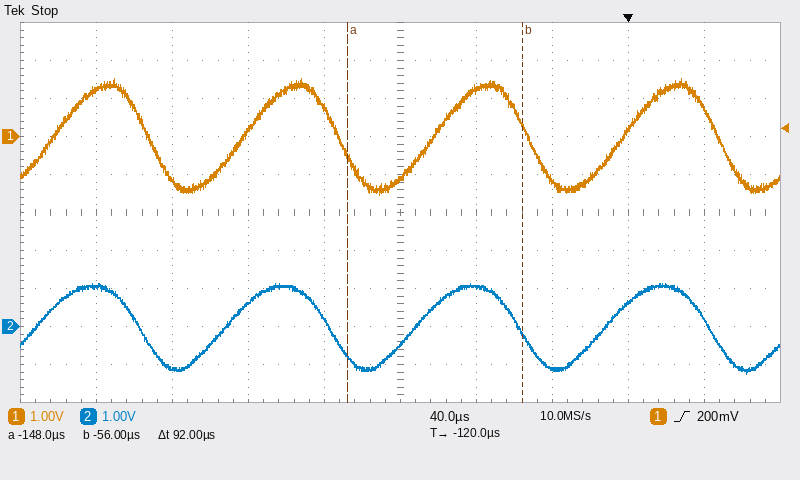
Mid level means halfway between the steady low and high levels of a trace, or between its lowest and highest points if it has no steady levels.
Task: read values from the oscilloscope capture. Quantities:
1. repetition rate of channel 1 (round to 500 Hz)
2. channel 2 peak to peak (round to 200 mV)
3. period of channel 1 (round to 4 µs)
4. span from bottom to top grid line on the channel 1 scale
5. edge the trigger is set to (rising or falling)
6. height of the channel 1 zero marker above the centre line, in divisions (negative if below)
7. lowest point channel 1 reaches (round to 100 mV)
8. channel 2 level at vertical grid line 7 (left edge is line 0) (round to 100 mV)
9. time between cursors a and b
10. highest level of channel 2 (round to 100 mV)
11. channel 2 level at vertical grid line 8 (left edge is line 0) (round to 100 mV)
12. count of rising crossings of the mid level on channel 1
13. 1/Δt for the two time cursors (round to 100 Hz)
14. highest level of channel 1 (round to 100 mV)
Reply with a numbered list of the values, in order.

1. 10.0 kHz
2. 2.4 V
3. 100 µs
4. 10 V
5. rising
6. +2.0 div
7. -1.5 V
8. -1.1 V
9. 92 µs
10. 1.1 V
11. 600 mV
12. 4
13. 10.9 kHz
14. 1.5 V
